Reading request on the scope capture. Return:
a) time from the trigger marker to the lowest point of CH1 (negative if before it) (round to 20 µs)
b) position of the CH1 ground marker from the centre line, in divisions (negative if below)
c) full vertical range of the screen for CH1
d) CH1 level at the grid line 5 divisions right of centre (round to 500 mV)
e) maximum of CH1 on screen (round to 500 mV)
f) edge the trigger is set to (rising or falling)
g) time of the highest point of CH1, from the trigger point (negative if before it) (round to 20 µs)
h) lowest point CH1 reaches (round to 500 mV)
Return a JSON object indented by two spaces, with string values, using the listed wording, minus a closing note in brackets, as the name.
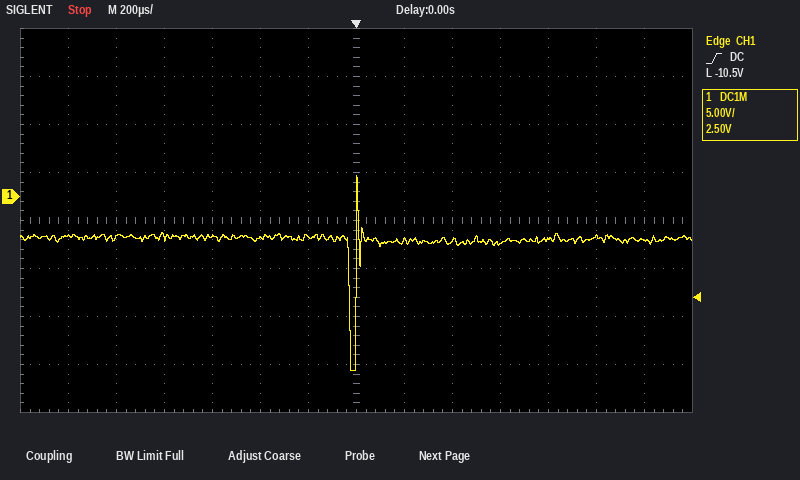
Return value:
{
  "time from the trigger marker to the lowest point of CH1 (negative if before it)": "-20 µs",
  "position of the CH1 ground marker from the centre line, in divisions": "+0.5 div",
  "full vertical range of the screen for CH1": "40 V",
  "CH1 level at the grid line 5 divisions right of centre": "-4.0 V",
  "maximum of CH1 on screen": "2.0 V",
  "edge the trigger is set to": "rising",
  "time of the highest point of CH1, from the trigger point (negative if before it)": "0 µs",
  "lowest point CH1 reaches": "-18.0 V"
}
